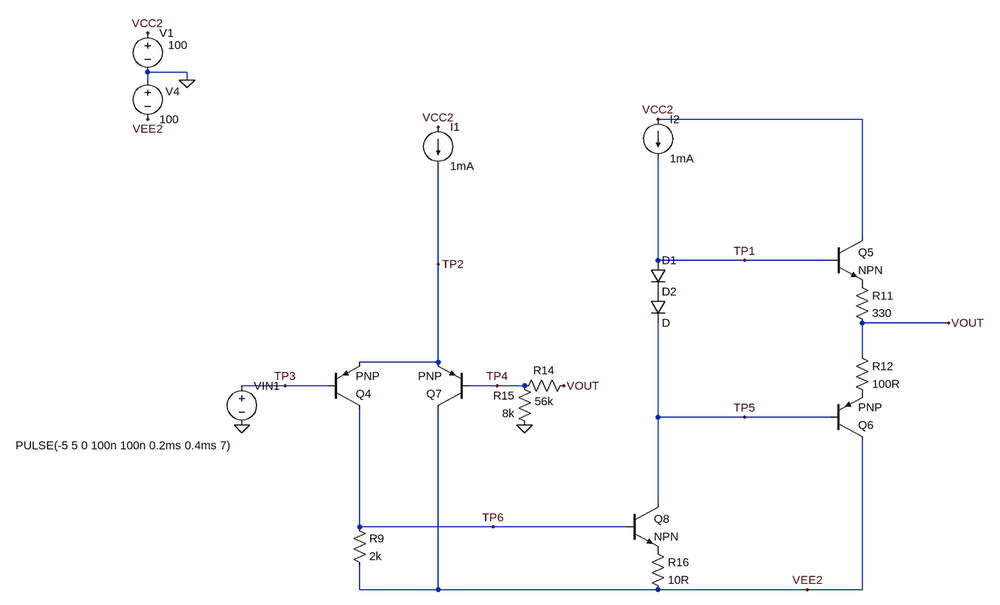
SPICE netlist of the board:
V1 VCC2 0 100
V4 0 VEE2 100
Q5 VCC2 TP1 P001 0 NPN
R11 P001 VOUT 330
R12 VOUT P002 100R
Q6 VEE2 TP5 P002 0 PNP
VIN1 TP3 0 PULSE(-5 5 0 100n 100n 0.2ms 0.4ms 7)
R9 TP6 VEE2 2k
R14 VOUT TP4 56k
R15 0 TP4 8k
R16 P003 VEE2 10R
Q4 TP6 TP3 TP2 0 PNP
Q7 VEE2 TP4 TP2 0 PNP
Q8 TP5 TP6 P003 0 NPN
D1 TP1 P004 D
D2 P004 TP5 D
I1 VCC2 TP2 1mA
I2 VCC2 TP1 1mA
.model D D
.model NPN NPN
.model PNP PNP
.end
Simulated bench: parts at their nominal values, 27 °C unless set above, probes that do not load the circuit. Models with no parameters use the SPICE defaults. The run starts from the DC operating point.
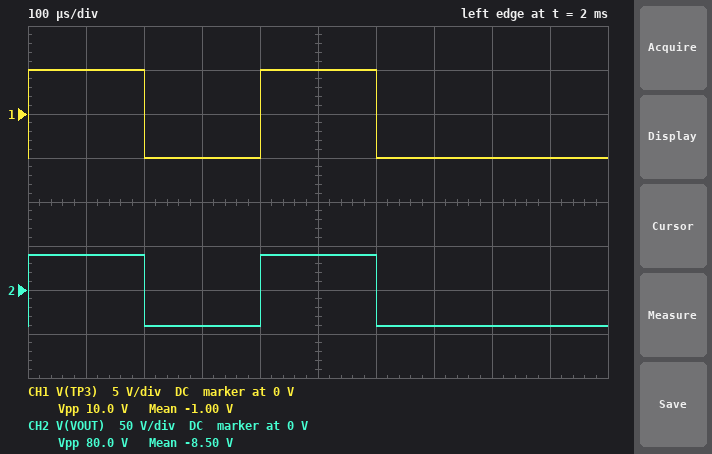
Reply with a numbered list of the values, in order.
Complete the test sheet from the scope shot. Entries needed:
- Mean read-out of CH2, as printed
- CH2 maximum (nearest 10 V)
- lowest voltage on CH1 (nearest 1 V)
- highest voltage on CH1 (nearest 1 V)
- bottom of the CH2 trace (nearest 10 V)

1. -8.50 V
2. 40 V
3. -5 V
4. 5 V
5. -40 V
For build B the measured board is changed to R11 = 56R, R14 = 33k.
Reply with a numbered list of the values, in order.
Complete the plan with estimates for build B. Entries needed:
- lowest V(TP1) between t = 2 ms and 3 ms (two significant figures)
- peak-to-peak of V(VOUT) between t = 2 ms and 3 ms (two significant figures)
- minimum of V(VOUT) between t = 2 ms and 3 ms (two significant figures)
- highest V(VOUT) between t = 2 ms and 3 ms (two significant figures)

1. -25 V
2. 51 V
3. -26 V
4. 25 V
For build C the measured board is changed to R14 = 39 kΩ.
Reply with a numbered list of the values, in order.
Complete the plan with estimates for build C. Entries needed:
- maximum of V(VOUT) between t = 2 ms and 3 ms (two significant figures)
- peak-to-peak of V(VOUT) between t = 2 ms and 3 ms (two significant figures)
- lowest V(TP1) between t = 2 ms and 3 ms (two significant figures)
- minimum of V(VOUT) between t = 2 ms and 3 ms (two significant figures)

1. 29 V
2. 59 V
3. -29 V
4. -30 V
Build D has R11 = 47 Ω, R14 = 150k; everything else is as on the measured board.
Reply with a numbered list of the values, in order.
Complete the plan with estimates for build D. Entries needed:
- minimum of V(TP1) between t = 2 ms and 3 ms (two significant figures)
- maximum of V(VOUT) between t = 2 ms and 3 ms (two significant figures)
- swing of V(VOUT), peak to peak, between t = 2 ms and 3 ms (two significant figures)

1. -99 V
2. 98 V
3. 200 V
